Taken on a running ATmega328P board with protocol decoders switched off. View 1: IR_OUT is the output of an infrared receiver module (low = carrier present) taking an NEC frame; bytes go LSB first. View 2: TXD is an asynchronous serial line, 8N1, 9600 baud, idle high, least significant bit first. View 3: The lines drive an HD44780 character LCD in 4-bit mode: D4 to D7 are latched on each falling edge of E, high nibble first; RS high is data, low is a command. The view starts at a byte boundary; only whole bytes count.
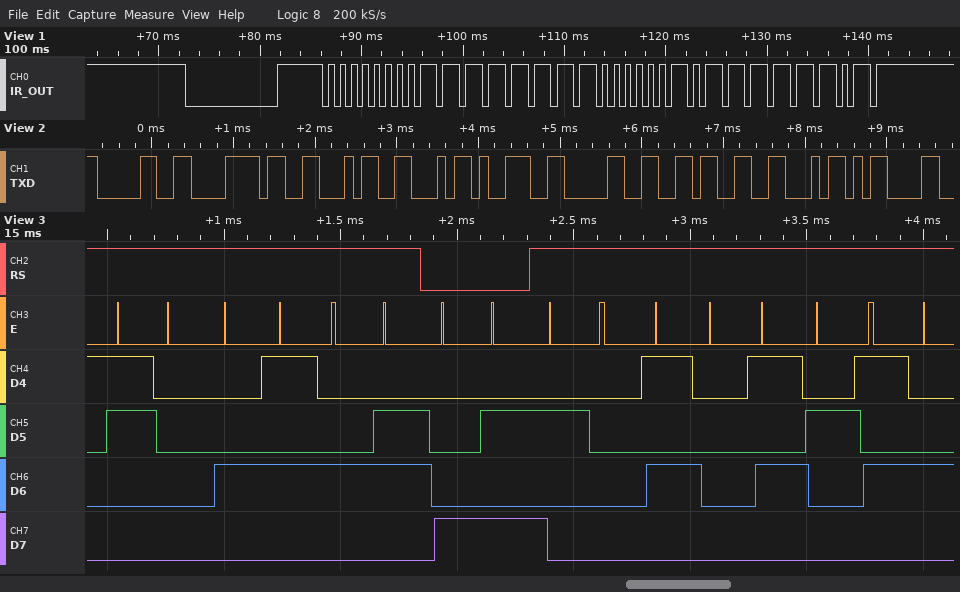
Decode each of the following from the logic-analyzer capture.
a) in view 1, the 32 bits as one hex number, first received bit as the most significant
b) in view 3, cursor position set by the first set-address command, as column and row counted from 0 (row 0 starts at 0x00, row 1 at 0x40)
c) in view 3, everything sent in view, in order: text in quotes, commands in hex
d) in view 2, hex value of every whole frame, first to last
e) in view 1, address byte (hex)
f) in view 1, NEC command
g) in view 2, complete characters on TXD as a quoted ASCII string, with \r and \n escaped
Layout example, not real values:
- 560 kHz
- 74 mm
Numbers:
- 0x00FF02FD
- column 10, row 0
- "0EF" 0x8A " PRT"
- 0x30 0x78 0x46 0x46 0x39 0x30 0x36 0x46 0x0D
- 0x00
- 0x40
- "0xFF906F\r"
